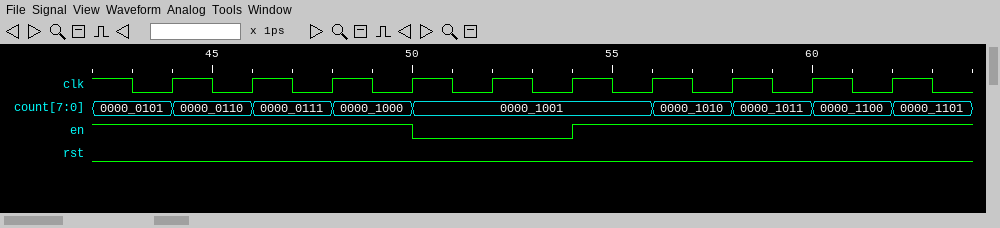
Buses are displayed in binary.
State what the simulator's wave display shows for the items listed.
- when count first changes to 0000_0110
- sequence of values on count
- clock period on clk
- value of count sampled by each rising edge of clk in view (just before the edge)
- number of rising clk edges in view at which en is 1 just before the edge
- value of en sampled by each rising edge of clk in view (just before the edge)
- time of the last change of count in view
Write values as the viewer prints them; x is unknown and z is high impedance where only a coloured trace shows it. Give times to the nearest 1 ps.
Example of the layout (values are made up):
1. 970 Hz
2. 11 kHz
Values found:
1. 44 ps
2. 0000_0101, 0000_0110, 0000_0111, 0000_1000, 0000_1001, 0000_1010, 0000_1011, 0000_1100, 0000_1101
3. 2 ps
4. 0000_0101, 0000_0110, 0000_0111, 0000_1000, 0000_1001, 0000_1001, 0000_1001, 0000_1010, 0000_1011, 0000_1100
5. 8
6. 1 1 1 1 0 0 1 1 1 1
7. 62 ps
